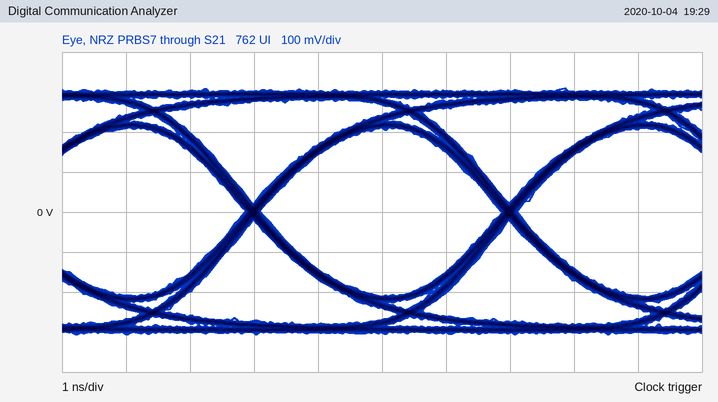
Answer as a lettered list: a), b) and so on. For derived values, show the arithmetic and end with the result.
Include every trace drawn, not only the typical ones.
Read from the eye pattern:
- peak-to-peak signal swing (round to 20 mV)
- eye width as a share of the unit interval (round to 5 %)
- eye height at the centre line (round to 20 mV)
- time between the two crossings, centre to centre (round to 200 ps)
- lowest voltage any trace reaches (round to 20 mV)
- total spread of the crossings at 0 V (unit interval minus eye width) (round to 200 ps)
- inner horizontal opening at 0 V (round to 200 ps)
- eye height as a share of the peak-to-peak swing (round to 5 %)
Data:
a) 620 mV
b) 3.8 ns / 4.0 ns ≈ 95 %
c) 420 mV
d) 4.0 ns
e) -300 mV
f) 200 ps
g) 3.8 ns
h) 420 mV / 620 mV ≈ 67.7 %, so 70 % to the nearest 5 %
